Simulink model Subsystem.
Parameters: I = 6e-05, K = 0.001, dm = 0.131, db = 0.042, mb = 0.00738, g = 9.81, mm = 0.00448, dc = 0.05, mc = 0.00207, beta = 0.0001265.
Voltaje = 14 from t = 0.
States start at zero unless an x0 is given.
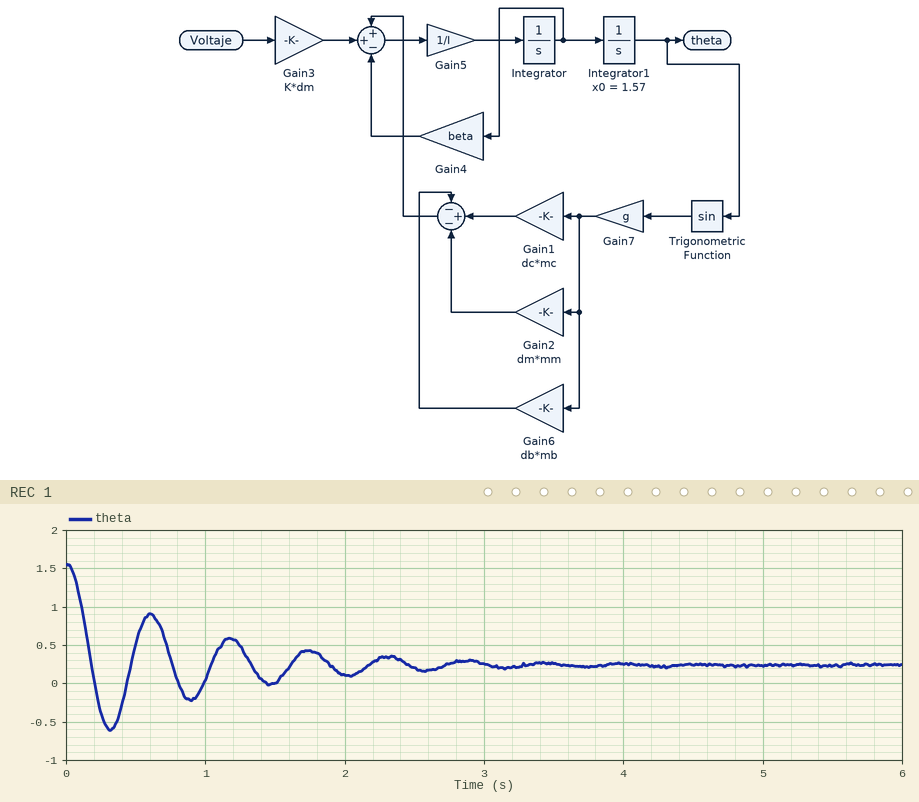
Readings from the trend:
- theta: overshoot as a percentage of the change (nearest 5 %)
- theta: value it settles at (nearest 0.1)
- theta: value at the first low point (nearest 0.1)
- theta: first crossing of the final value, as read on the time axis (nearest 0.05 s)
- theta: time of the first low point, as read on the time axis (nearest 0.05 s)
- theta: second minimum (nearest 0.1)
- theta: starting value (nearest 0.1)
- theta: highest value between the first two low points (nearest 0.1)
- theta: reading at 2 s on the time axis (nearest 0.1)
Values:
65 %
0.2
-0.6
0.20 s
0.30 s
-0.2
1.6
0.9
0.1
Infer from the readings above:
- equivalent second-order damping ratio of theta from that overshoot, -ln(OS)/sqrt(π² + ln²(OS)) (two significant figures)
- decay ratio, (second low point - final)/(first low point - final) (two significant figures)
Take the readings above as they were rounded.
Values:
0.14
0.50
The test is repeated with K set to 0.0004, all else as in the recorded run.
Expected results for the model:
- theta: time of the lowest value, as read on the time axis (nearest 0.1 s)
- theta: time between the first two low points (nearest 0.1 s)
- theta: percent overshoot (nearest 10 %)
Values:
0.3 s
0.6 s
70 %
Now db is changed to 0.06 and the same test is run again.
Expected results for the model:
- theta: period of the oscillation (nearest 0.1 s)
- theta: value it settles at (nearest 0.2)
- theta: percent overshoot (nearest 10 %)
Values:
0.5 s
0.2
70 %
